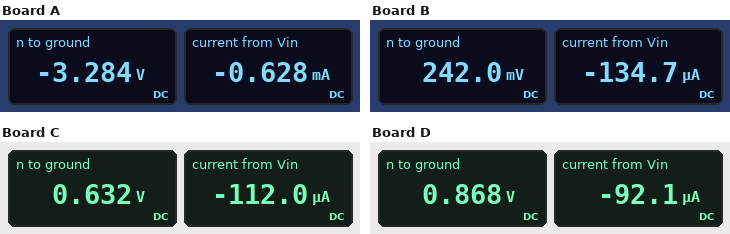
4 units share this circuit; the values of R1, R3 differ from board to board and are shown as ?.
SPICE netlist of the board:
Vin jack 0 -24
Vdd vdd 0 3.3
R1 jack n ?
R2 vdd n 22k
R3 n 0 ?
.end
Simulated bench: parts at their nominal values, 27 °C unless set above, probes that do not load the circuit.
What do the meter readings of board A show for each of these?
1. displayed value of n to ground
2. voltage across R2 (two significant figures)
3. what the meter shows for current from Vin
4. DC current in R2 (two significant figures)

-3.284 V
6.6 V
-0.628 mA
300 µA
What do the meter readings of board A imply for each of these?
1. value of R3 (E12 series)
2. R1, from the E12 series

10 kΩ
33 kΩ
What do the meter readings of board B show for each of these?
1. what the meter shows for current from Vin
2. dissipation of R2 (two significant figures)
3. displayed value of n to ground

-134.7 µA
430 µW
242.0 mV
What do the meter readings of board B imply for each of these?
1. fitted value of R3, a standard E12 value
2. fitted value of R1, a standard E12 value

56 kΩ
180 kΩ
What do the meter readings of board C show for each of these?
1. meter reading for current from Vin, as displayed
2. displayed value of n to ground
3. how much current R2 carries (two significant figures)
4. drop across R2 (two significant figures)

-112.0 µA
0.632 V
120 µA
2.7 V
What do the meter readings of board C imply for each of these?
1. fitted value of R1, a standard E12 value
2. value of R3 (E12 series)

220 kΩ
68 kΩ
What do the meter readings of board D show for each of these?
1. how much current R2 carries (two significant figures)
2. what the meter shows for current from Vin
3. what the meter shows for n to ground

110 µA
-92.1 µA
0.868 V
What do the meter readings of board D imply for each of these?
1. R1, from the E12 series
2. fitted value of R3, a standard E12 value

270 kΩ
47 kΩ
